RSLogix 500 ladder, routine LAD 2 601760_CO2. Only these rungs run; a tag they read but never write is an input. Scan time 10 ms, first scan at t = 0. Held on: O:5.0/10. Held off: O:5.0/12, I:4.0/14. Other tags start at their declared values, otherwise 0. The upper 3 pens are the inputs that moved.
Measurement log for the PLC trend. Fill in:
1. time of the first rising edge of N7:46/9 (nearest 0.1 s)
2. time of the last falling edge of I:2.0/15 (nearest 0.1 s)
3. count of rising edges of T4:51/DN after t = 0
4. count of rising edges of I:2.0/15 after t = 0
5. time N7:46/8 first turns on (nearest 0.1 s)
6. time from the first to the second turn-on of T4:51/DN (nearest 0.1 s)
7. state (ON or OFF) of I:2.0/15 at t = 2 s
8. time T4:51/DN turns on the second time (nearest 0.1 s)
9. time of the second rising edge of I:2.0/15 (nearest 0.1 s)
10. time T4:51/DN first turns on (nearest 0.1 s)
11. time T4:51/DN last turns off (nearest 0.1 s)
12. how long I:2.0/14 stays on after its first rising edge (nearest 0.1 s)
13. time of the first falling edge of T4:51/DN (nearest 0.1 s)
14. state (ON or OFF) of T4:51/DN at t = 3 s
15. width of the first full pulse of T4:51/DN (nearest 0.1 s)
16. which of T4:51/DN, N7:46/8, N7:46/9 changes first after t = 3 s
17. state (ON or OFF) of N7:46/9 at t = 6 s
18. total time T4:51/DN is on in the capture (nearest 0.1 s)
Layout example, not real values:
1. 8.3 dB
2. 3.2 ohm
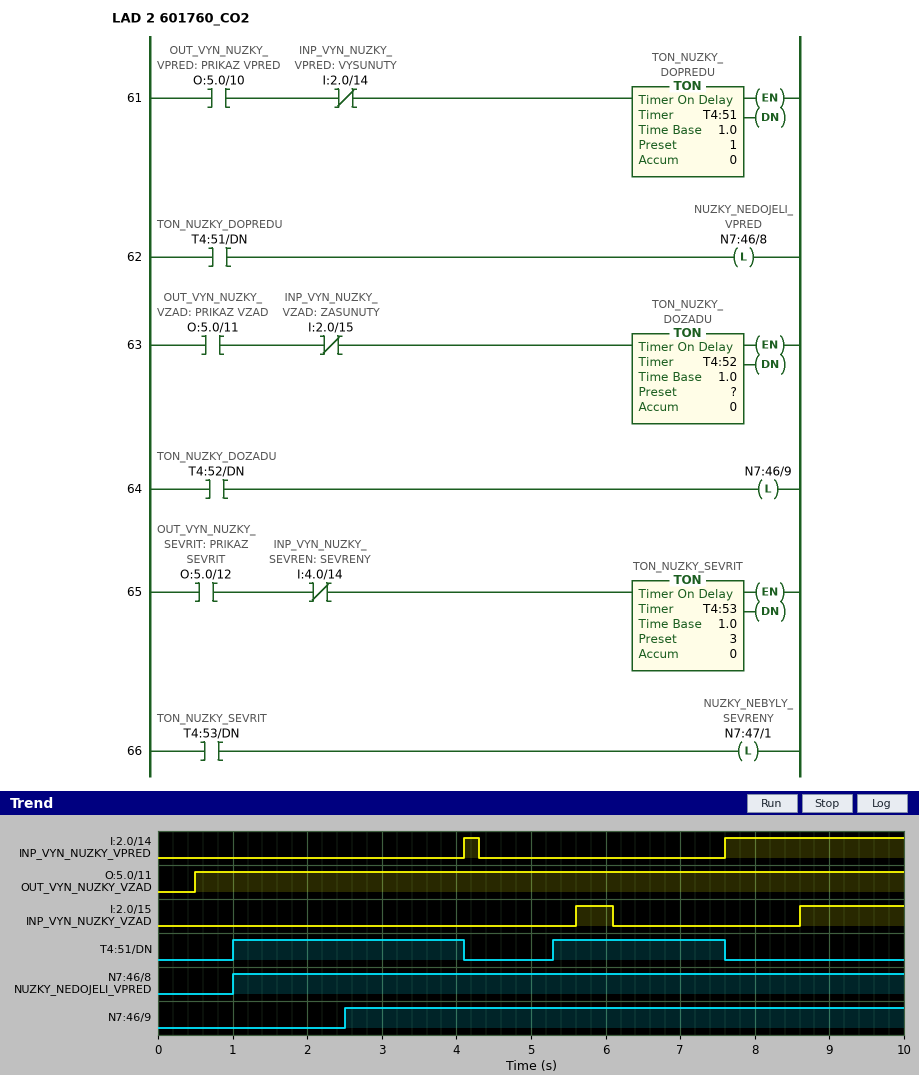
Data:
1. 2.5 s
2. 6.1 s
3. 2
4. 2
5. 1.0 s
6. 4.3 s
7. OFF
8. 5.3 s
9. 8.6 s
10. 1.0 s
11. 7.6 s
12. 0.2 s
13. 4.1 s
14. ON
15. 3.1 s
16. T4:51/DN
17. ON
18. 5.4 s
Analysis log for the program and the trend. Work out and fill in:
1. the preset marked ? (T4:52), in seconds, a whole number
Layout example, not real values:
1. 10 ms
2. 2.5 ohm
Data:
1. 2 s
